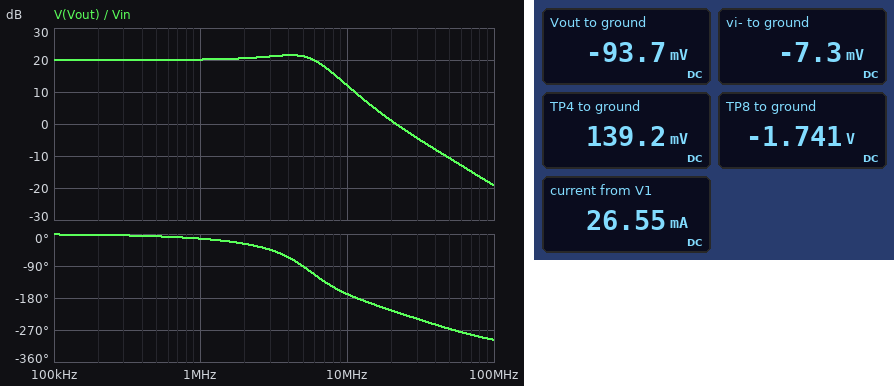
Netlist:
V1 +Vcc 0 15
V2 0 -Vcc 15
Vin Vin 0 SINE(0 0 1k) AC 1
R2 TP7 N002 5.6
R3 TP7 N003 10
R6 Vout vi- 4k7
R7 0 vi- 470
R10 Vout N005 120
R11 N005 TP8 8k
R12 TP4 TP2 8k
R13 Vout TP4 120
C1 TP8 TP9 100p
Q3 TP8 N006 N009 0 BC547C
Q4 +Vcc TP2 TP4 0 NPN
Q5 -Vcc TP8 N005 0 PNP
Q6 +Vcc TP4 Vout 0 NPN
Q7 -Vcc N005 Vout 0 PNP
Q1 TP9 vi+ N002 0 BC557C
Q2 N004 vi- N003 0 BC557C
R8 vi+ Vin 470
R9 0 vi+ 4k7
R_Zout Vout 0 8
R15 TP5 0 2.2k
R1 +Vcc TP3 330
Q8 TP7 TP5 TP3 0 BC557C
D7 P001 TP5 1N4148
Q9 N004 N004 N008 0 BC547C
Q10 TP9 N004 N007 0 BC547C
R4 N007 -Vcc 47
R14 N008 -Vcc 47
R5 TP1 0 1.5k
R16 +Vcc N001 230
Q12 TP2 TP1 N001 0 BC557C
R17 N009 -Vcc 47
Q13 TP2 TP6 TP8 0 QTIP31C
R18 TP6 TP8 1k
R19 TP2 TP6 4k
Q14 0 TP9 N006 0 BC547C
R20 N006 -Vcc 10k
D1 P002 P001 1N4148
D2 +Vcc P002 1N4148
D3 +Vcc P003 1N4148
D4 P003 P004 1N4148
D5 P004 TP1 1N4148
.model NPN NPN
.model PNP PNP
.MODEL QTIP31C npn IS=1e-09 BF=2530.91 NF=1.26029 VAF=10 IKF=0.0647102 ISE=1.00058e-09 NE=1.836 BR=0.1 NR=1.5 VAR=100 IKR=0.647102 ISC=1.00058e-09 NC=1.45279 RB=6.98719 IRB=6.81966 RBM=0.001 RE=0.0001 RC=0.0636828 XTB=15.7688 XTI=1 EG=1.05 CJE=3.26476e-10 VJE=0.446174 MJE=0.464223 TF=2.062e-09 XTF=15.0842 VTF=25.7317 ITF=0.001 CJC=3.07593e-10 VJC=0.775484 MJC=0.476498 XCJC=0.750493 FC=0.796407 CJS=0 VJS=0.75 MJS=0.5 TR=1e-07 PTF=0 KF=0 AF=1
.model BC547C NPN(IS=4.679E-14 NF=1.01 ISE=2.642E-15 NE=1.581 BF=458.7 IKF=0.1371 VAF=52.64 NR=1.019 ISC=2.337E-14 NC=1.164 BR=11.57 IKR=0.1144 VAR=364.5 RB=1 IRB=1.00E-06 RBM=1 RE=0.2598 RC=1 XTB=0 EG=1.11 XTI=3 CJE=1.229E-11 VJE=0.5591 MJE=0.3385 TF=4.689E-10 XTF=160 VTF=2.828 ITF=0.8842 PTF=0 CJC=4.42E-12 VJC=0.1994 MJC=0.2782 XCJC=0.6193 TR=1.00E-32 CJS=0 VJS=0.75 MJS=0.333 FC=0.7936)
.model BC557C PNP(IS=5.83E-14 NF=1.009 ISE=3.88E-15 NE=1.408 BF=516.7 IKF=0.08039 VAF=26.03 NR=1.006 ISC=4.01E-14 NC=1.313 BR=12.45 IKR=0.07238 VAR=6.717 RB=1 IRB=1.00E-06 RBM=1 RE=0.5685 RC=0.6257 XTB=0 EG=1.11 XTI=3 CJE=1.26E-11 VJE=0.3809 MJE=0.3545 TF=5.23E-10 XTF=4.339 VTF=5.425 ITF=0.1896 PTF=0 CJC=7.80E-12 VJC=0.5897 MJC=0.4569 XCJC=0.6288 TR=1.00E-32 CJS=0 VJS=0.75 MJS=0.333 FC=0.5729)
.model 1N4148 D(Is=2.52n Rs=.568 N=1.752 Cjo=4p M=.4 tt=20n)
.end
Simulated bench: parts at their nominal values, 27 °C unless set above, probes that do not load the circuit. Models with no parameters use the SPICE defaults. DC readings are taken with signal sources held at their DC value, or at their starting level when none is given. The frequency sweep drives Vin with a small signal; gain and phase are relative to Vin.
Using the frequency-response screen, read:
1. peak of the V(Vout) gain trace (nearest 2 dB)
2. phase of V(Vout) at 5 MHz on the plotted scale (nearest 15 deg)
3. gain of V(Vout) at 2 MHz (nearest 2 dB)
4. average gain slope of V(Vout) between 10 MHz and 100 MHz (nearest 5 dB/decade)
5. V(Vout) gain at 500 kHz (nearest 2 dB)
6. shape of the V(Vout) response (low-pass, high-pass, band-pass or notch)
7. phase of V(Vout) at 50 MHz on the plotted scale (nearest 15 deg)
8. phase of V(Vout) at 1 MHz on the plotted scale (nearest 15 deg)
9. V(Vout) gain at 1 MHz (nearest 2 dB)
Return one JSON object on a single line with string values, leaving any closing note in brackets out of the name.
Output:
{"peak of the V(Vout) gain trace": "22 dB", "phase of V(Vout) at 5 MHz on the plotted scale": "-90 deg", "gain of V(Vout) at 2 MHz": "20 dB", "average gain slope of V(Vout) between 10 MHz and 100 MHz": "-30 dB/decade", "V(Vout) gain at 500 kHz": "20 dB", "shape of the V(Vout) response": "low-pass", "phase of V(Vout) at 50 MHz on the plotted scale": "-270 deg", "phase of V(Vout) at 1 MHz on the plotted scale": "-15 deg", "V(Vout) gain at 1 MHz": "20 dB"}
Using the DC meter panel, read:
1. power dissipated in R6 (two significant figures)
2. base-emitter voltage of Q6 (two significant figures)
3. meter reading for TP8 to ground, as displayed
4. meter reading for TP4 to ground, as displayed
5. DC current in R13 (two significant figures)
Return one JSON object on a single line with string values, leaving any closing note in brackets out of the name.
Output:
{"power dissipated in R6": "1.6 µW", "base-emitter voltage of Q6": "230 mV", "meter reading for TP8 to ground, as displayed": "-1.741 V", "meter reading for TP4 to ground, as displayed": "139.2 mV", "DC current in R13": "1.9 mA"}
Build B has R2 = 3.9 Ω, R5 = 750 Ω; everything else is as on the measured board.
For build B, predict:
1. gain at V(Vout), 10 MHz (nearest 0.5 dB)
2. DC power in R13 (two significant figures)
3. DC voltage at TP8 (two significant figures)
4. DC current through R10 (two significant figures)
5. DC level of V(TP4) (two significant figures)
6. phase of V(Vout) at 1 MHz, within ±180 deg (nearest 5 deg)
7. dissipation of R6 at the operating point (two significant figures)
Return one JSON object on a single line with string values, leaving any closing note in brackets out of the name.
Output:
{"gain at V(Vout), 10 MHz": "14.0 dB", "DC power in R13": "480 µW", "DC voltage at TP8": "-1.8 V", "DC current through R10": "7.0 mA", "DC level of V(TP4)": "110 mV", "phase of V(Vout) at 1 MHz, within ±180 deg": "-10 deg", "dissipation of R6 at the operating point": "3.1 µW"}
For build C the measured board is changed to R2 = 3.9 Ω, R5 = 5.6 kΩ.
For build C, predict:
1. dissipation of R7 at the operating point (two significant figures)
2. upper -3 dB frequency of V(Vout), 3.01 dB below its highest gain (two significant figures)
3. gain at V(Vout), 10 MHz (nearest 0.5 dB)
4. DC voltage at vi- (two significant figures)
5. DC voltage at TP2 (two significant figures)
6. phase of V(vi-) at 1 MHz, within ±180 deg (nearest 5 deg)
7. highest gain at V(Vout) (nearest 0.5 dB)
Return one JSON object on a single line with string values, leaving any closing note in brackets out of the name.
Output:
{"dissipation of R7 at the operating point": "250 nW", "upper -3 dB frequency of V(Vout), 3.01 dB below its highest gain": "7.2 MHz", "gain at V(Vout), 10 MHz": "14.0 dB", "DC voltage at vi-": "-11 mV", "DC voltage at TP2": "830 mV", "phase of V(vi-) at 1 MHz, within ±180 deg": "-10 deg", "highest gain at V(Vout)": "22.5 dB"}
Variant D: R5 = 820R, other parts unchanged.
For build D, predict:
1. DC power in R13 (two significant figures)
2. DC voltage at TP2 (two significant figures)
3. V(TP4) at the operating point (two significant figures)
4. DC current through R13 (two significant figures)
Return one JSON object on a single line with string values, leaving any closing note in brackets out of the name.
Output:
{"DC power in R13": "520 µW", "DC voltage at TP2": "950 mV", "V(TP4) at the operating point": "160 mV", "DC current through R13": "2.1 mA"}
